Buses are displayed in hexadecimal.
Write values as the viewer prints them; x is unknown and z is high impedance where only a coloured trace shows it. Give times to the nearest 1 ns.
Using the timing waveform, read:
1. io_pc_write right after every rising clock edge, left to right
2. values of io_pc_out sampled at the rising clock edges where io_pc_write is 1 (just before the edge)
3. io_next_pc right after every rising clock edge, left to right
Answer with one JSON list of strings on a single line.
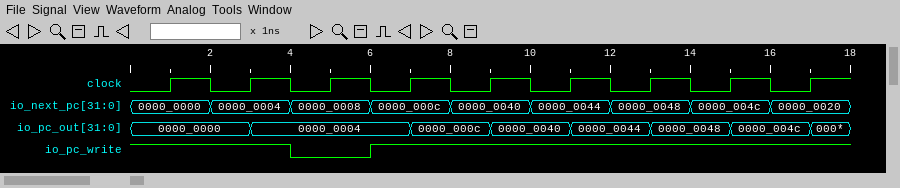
["1 1 0 1 1 1 1 1 1", "0000_0000, 0000_0000, 0000_0004, 0000_000c, 0000_0040, 0000_0044, 0000_0048, 0000_004c", "0000_0000, 0000_0004, 0000_0008, 0000_000c, 0000_0040, 0000_0044, 0000_0048, 0000_004c, 0000_0020"]
